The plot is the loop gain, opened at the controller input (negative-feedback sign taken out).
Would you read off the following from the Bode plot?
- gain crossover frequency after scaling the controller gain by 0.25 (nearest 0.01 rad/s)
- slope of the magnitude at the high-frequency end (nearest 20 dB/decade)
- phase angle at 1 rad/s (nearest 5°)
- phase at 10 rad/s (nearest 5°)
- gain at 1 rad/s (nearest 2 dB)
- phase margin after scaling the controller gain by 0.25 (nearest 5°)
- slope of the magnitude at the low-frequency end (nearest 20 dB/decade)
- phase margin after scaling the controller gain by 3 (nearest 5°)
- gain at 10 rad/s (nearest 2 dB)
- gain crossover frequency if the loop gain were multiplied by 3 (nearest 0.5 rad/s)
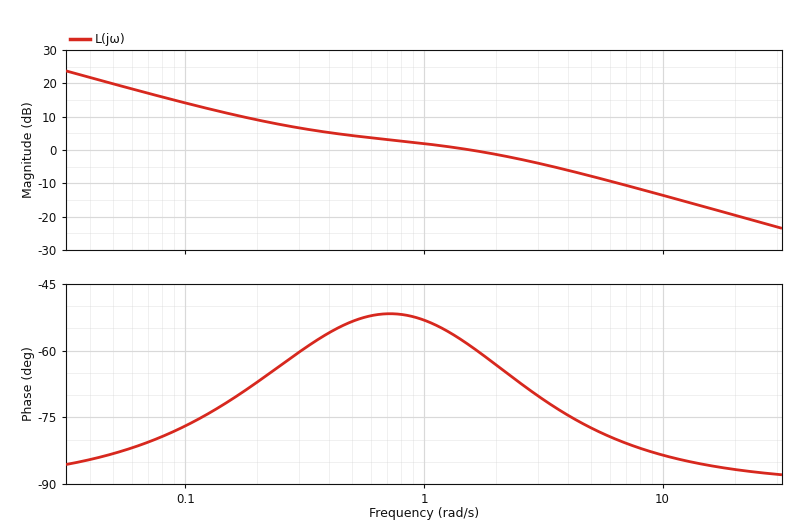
0.13 rad/s
-20 dB/decade
-55°
-85°
2 dB
105°
-20 dB/decade
100°
-14 dB
6.0 rad/s
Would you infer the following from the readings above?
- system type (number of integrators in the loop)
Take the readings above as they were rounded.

1
